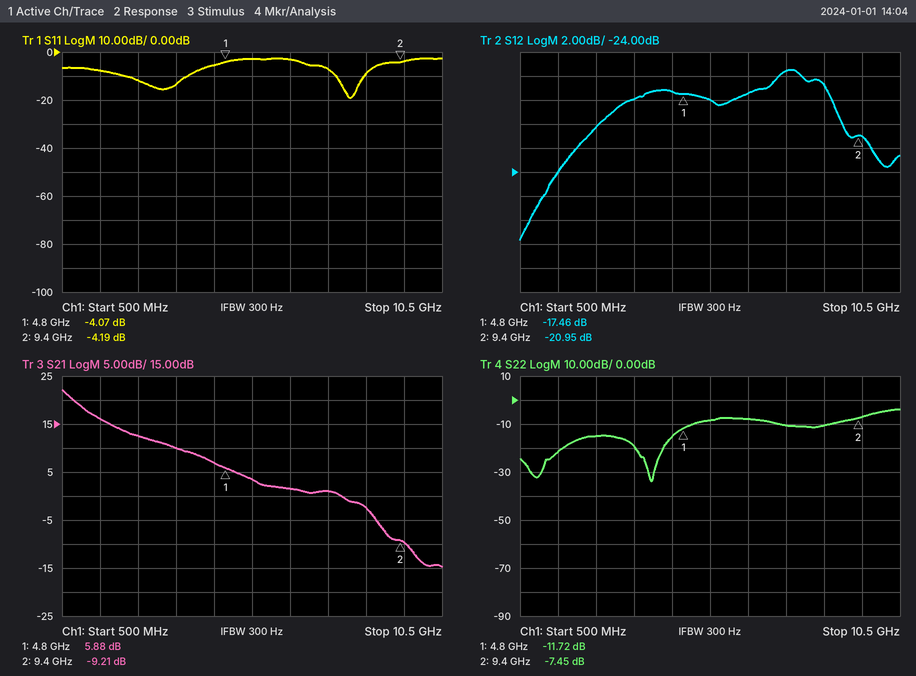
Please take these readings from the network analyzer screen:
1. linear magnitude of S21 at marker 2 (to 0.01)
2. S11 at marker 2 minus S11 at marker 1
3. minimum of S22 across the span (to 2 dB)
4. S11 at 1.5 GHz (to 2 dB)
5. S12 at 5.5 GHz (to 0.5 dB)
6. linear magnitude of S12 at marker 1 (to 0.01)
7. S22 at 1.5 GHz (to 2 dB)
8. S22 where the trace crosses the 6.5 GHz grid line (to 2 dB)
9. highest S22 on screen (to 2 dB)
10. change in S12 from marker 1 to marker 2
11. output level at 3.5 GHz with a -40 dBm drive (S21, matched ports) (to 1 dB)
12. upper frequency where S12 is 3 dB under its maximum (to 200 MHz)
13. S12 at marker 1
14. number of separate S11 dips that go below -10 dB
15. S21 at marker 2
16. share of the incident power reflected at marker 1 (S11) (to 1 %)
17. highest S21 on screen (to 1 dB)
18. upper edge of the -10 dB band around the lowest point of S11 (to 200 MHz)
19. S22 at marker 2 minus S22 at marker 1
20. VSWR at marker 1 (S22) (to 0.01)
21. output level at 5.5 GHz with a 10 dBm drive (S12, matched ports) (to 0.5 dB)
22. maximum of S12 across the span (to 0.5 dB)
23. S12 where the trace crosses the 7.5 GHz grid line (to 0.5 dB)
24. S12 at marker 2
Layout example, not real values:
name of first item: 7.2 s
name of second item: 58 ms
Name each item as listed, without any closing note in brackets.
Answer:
linear magnitude of S21 at marker 2: 0.35
S11 at marker 2 minus S11 at marker 1: -0.12 dB
minimum of S22 across the span: -34 dB
S11 at 1.5 GHz: -8 dB
S12 at 5.5 GHz: -18.0 dB
linear magnitude of S12 at marker 1: 0.13
S22 at 1.5 GHz: -22 dB
S22 where the trace crosses the 6.5 GHz grid line: -8 dB
highest S22 on screen: -4 dB
change in S12 from marker 1 to marker 2: -3.49 dB
output level at 3.5 GHz with a -40 dBm drive (S21, matched ports): -30 dBm
upper frequency where S12 is 3 dB under its maximum: 8.8 GHz
S12 at marker 1: -17.46 dB
number of separate S11 dips that go below -10 dB: 2
S21 at marker 2: -9.21 dB
share of the incident power reflected at marker 1 (S11): 39 %
highest S21 on screen: 22 dB
upper edge of the -10 dB band around the lowest point of S11: 8.4 GHz
S22 at marker 2 minus S22 at marker 1: 4.27 dB
VSWR at marker 1 (S22): 1.70
output level at 5.5 GHz with a 10 dBm drive (S12, matched ports): -8.0 dBm
maximum of S12 across the span: -15.5 dB
S12 where the trace crosses the 7.5 GHz grid line: -15.5 dB
S12 at marker 2: -20.95 dB
